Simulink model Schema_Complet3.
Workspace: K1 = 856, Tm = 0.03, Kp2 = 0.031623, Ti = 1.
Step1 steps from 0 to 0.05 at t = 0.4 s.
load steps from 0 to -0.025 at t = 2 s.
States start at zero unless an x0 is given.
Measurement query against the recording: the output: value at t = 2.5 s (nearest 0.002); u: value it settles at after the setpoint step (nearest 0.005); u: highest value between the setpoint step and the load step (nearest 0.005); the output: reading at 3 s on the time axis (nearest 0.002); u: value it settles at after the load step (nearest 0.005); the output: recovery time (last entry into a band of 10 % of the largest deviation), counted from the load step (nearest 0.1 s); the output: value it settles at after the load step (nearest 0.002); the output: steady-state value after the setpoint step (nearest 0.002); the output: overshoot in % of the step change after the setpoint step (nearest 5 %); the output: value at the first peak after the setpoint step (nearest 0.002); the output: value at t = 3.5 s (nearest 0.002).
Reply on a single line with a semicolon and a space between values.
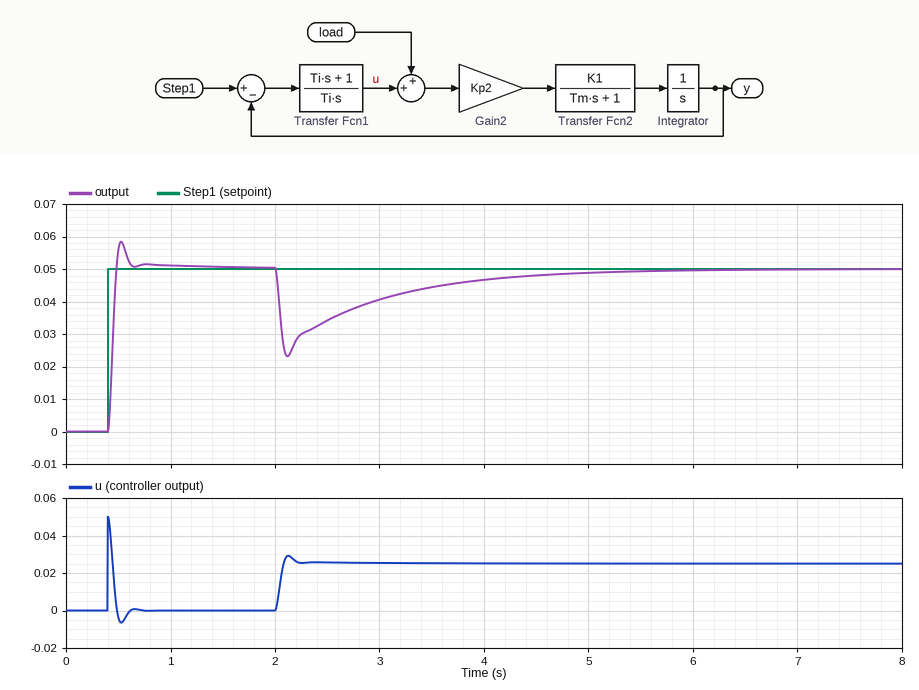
0.034; 0.000; 0.050; 0.040; 0.025; 2.2 s; 0.050; 0.050; 15 %; 0.058; 0.044
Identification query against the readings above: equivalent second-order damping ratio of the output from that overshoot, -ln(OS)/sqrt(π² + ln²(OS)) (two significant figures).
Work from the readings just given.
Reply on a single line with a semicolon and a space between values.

0.52
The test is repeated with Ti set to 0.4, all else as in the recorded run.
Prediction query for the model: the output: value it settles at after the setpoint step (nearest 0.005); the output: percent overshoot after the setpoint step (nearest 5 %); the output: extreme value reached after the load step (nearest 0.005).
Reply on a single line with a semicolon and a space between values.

0.050; 25 %; 0.025
